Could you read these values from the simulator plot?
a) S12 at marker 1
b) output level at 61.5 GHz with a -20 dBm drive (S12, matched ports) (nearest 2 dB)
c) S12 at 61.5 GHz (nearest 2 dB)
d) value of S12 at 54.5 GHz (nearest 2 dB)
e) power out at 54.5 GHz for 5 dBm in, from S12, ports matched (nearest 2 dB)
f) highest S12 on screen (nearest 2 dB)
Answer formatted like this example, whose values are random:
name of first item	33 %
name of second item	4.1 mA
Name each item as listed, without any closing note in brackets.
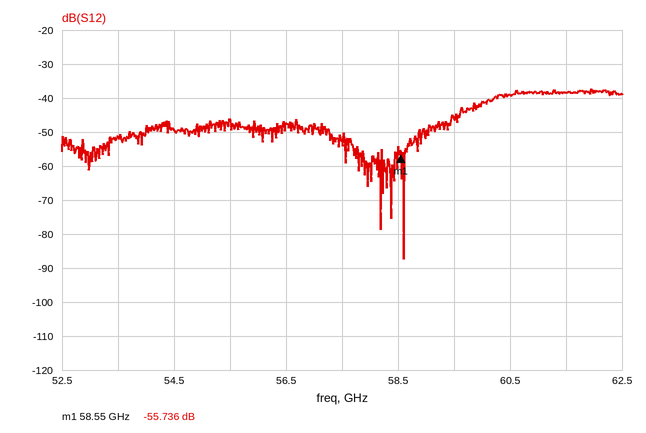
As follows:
S12 at marker 1	-55.736 dB
output level at 61.5 GHz with a -20 dBm drive (S12, matched ports)	-58 dBm
S12 at 61.5 GHz	-38 dB
value of S12 at 54.5 GHz	-50 dB
power out at 54.5 GHz for 5 dBm in, from S12, ports matched	-44 dBm
highest S12 on screen	-38 dB
